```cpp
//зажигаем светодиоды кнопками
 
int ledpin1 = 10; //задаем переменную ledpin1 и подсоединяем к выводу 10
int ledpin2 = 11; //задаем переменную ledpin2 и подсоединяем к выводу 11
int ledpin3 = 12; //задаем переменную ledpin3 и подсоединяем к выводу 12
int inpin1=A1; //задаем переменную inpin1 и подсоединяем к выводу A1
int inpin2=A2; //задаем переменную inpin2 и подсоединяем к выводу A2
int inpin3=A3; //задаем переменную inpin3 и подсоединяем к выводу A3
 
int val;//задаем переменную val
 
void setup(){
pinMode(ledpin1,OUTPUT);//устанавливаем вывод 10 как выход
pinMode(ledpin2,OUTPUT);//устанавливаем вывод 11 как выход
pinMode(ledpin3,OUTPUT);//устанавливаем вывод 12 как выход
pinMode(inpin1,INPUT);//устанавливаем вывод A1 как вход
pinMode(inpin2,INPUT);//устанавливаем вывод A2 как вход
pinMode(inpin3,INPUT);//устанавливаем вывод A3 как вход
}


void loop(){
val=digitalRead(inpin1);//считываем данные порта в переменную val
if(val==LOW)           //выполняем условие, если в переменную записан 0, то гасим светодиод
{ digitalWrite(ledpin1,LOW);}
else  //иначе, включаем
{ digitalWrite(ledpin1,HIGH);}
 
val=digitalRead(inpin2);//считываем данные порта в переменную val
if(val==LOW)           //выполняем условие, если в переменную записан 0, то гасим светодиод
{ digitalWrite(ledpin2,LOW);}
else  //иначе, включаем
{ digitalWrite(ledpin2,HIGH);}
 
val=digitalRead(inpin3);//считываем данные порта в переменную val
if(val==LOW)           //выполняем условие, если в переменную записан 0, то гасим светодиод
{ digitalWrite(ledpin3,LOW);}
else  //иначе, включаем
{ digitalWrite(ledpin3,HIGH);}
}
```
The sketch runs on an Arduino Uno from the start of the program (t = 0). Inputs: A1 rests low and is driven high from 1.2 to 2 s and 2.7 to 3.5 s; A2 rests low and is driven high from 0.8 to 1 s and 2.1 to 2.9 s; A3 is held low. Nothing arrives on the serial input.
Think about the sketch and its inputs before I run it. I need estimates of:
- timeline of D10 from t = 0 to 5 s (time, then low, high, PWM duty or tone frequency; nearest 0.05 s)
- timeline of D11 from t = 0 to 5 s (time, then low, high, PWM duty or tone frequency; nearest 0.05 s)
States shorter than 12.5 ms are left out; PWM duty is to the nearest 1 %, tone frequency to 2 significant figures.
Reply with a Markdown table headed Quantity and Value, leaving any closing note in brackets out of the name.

| Quantity | Value |
|---|---|
| timeline of D10 from t = 0 to 5 s | 0 s low; 1.2 s high; 2 s low; 2.7 s high; 3.5 s low |
| timeline of D11 from t = 0 to 5 s | 0 s low; 0.8 s high; 1 s low; 2.1 s high; 2.9 s low |
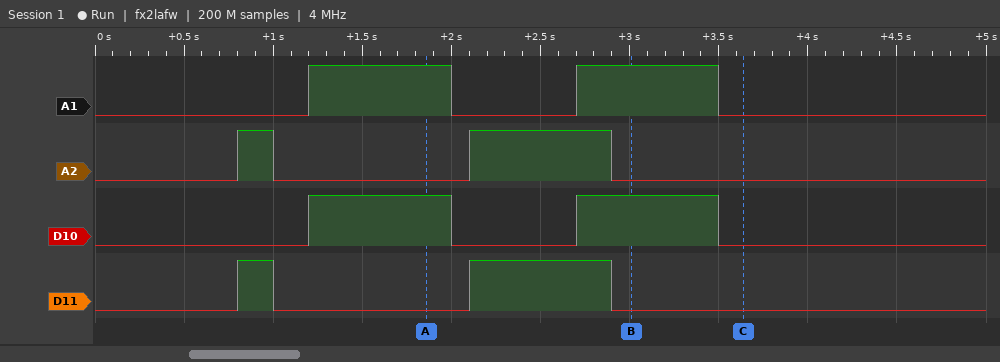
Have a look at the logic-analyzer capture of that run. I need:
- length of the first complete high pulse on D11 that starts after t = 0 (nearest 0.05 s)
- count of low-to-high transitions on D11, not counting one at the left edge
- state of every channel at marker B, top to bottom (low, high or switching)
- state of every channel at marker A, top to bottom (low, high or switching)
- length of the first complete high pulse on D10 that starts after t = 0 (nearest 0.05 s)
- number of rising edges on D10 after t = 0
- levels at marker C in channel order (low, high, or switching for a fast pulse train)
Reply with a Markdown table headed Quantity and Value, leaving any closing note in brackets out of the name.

| Quantity | Value |
|---|---|
| length of the first complete high pulse on D11 that starts after t = 0 | 0.20 s |
| count of low-to-high transitions on D11, not counting one at the left edge | 2 |
| state of every channel at marker B, top to bottom | A1 high, A2 low, D10 high, D11 low |
| state of every channel at marker A, top to bottom | A1 high, A2 low, D10 high, D11 low |
| length of the first complete high pulse on D10 that starts after t = 0 | 0.80 s |
| number of rising edges on D10 after t = 0 | 2 |
| levels at marker C in channel order | A1 low, A2 low, D10 low, D11 low |
